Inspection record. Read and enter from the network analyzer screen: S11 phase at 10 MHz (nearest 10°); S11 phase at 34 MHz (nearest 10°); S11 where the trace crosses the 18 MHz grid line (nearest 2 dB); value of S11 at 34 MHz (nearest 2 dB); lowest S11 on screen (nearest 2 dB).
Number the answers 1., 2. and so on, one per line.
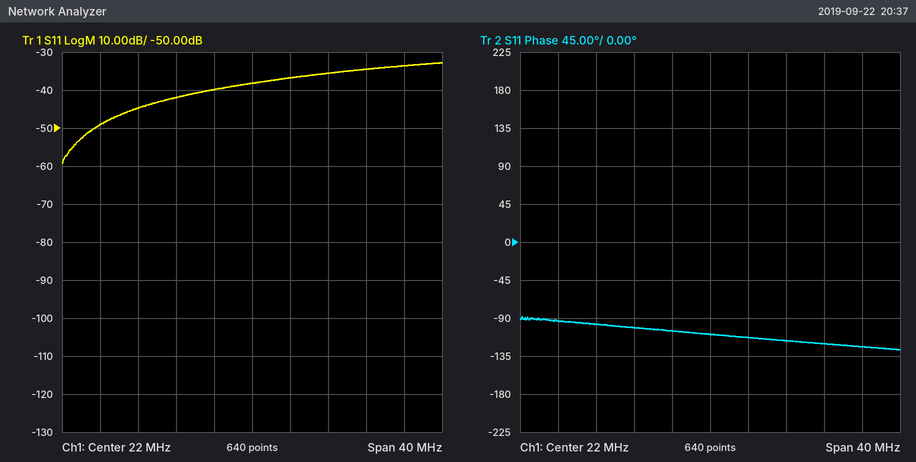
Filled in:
1. -100°
2. -120°
3. -40 dB
4. -34 dB
5. -60 dB
